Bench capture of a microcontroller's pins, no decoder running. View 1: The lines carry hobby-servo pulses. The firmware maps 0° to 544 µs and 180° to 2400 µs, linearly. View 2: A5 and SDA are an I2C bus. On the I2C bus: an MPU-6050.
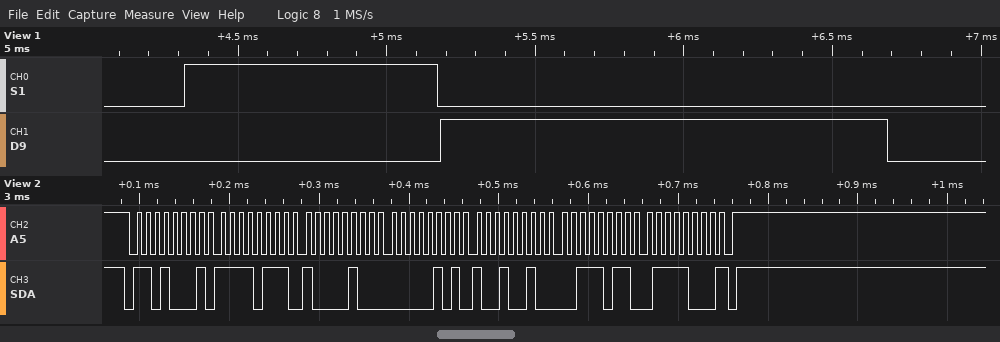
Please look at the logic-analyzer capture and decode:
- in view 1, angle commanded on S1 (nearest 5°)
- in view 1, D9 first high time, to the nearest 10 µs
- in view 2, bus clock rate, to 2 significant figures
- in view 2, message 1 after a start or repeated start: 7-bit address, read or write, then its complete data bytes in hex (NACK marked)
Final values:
30°
1500 µs
100 kHz
0x68 read: F7 84 05 92 3B 78 NACK
